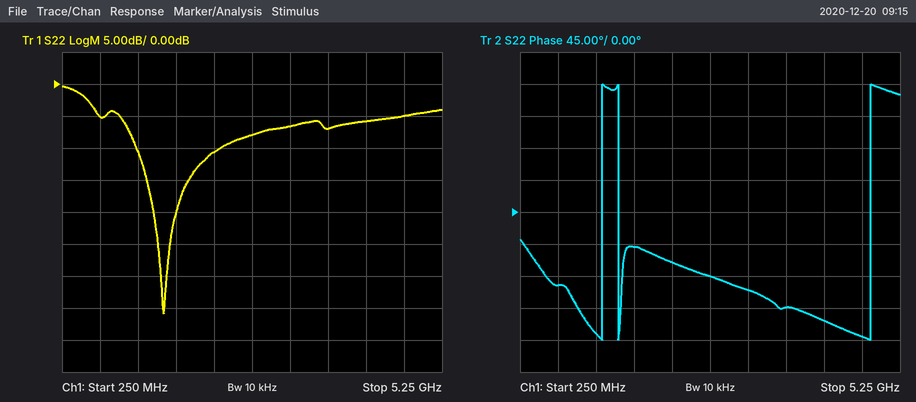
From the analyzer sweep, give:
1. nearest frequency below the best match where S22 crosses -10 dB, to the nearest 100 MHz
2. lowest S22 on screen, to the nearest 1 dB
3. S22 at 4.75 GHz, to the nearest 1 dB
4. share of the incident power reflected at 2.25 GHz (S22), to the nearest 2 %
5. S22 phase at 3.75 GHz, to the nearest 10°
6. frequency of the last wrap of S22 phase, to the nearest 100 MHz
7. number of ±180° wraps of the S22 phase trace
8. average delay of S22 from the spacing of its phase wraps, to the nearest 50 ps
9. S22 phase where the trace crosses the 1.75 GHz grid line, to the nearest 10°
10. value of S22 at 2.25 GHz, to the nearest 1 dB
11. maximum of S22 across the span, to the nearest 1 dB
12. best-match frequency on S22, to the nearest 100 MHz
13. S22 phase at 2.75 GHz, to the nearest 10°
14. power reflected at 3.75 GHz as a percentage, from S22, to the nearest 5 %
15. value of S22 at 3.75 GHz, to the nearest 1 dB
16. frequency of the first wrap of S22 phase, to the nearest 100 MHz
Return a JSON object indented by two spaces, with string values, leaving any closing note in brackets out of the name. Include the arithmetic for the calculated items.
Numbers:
{
  "nearest frequency below the best match where S22 crosses -10 dB, to the nearest 100 MHz": "1.2 GHz",
  "lowest S22 on screen, to the nearest 1 dB": "-36 dB",
  "S22 at 4.75 GHz, to the nearest 1 dB": "-5 dB",
  "share of the incident power reflected at 2.25 GHz (S22), to the nearest 2 %": "10^(-11/10) ≈ 8 %",
  "S22 phase at 3.75 GHz, to the nearest 10°": "-130°",
  "frequency of the last wrap of S22 phase, to the nearest 100 MHz": "4.9 GHz",
  "number of ±180° wraps of the S22 phase trace": "3",
  "average delay of S22 from the spacing of its phase wraps, to the nearest 50 ps": "2 cycles / (4.9 GHz − 1.3 GHz) ≈ 556 ps, so 550 ps to the nearest 50 ps",
  "S22 phase where the trace crosses the 1.75 GHz grid line, to the nearest 10°": "-50°",
  "value of S22 at 2.25 GHz, to the nearest 1 dB": "-11 dB",
  "maximum of S22 across the span, to the nearest 1 dB": "0 dB",
  "best-match frequency on S22, to the nearest 100 MHz": "1.6 GHz",
  "S22 phase at 2.75 GHz, to the nearest 10°": "-90°",
  "power reflected at 3.75 GHz as a percentage, from S22, to the nearest 5 %": "10^(-7/10) ≈ 20 %",
  "value of S22 at 3.75 GHz, to the nearest 1 dB": "-7 dB",
  "frequency of the first wrap of S22 phase, to the nearest 100 MHz": "1.3 GHz"
}
